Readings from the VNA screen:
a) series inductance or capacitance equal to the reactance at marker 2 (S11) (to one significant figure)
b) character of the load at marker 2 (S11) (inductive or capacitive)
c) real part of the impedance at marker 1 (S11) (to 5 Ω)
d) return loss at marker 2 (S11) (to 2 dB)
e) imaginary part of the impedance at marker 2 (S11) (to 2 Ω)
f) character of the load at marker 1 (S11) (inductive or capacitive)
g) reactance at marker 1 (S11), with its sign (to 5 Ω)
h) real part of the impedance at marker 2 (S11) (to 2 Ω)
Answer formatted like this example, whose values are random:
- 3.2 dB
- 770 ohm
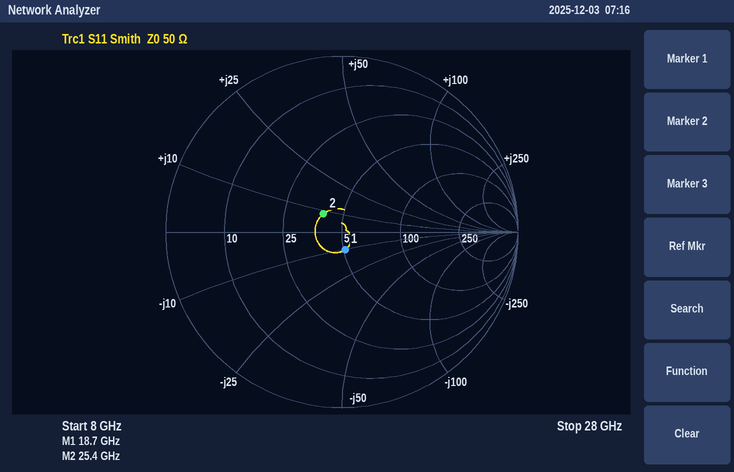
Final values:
- 50 pH
- inductive
- 50 Ω
- 16 dB
- +8 Ω
- capacitive
- -10 Ω
- 40 Ω
